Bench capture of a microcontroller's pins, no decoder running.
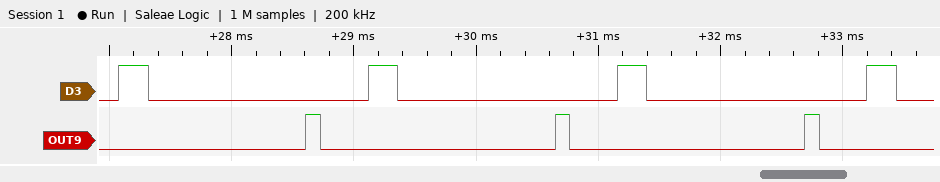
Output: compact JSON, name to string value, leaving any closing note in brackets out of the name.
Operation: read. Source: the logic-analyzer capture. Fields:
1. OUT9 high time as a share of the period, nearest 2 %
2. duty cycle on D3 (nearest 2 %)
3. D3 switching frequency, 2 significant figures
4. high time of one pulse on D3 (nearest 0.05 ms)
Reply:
{"OUT9 high time as a share of the period, nearest 2 %": "6 %", "duty cycle on D3": "12 %", "D3 switching frequency, 2 significant figures": "490 Hz", "high time of one pulse on D3": "0.25 ms"}
